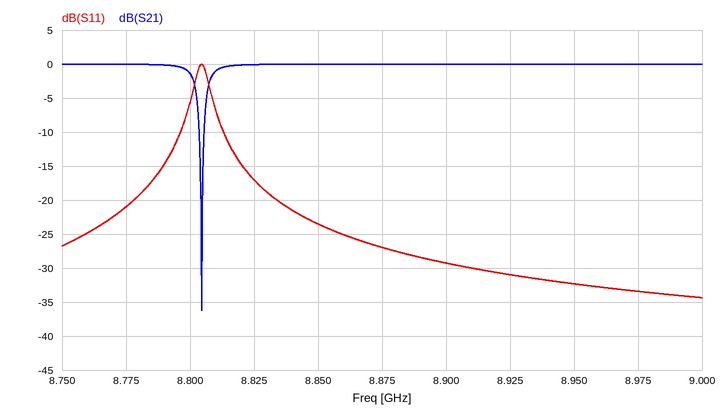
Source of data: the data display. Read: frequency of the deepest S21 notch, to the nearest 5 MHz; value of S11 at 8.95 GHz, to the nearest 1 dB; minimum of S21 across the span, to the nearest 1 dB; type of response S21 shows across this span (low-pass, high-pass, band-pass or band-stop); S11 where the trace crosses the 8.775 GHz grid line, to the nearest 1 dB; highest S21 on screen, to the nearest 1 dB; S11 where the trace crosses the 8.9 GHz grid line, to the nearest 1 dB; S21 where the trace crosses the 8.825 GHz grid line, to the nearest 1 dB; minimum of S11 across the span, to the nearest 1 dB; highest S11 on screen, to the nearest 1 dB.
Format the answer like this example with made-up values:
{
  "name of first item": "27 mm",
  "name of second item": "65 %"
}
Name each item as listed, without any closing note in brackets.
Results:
{
  "frequency of the deepest S21 notch, to the nearest 5 MHz": "8.805 GHz",
  "value of S11 at 8.95 GHz, to the nearest 1 dB": "-32 dB",
  "minimum of S21 across the span, to the nearest 1 dB": "-36 dB",
  "type of response S21 shows across this span": "band-stop",
  "S11 where the trace crosses the 8.775 GHz grid line, to the nearest 1 dB": "-21 dB",
  "highest S21 on screen, to the nearest 1 dB": "0 dB",
  "S11 where the trace crosses the 8.9 GHz grid line, to the nearest 1 dB": "-29 dB",
  "S21 where the trace crosses the 8.825 GHz grid line, to the nearest 1 dB": "0 dB",
  "minimum of S11 across the span, to the nearest 1 dB": "-34 dB",
  "highest S11 on screen, to the nearest 1 dB": "0 dB"
}
